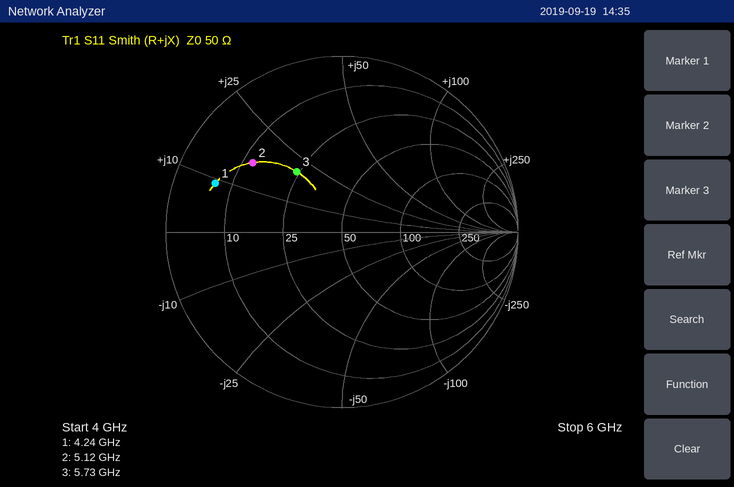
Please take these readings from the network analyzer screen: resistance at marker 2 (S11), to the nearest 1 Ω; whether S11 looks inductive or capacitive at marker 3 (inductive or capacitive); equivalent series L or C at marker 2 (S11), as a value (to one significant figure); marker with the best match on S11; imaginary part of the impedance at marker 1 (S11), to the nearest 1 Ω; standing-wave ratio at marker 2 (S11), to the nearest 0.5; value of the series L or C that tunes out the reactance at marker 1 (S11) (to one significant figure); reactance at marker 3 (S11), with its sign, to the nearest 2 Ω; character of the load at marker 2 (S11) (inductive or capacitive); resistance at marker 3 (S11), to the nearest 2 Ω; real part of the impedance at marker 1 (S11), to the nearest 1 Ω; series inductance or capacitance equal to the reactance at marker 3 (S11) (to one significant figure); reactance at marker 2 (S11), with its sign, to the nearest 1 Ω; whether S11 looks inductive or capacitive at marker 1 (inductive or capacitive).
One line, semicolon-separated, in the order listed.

12 Ω; inductive; 500 pH; marker 3; +9 Ω; 4.5; 4 pF; +20 Ω; inductive; 24 Ω; 7 Ω; 600 pH; +16 Ω; inductive
